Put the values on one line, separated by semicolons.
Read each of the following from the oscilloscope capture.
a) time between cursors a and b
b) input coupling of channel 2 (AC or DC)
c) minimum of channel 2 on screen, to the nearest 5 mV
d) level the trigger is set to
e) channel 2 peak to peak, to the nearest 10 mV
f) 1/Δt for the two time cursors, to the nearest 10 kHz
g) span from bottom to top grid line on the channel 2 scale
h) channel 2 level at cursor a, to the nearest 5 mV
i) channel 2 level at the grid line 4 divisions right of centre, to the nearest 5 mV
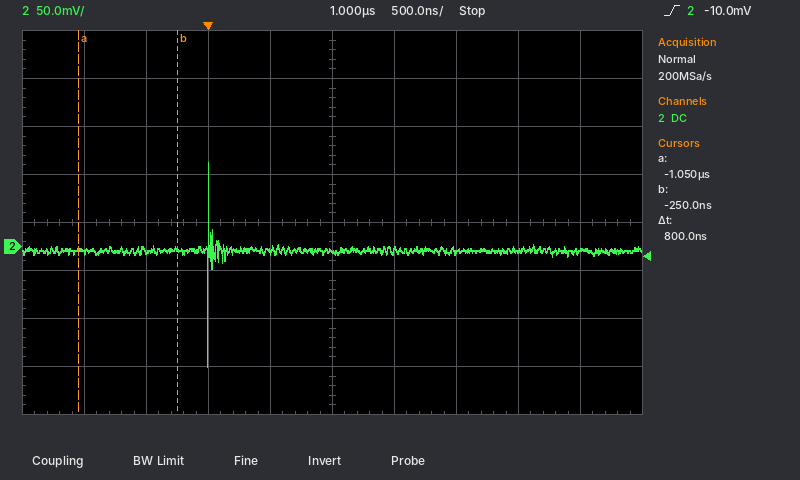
800 ns; DC; -125 mV; -10.0 mV; 210 mV; 1.25 MHz; 400 mV; -5 mV; -5 mV
